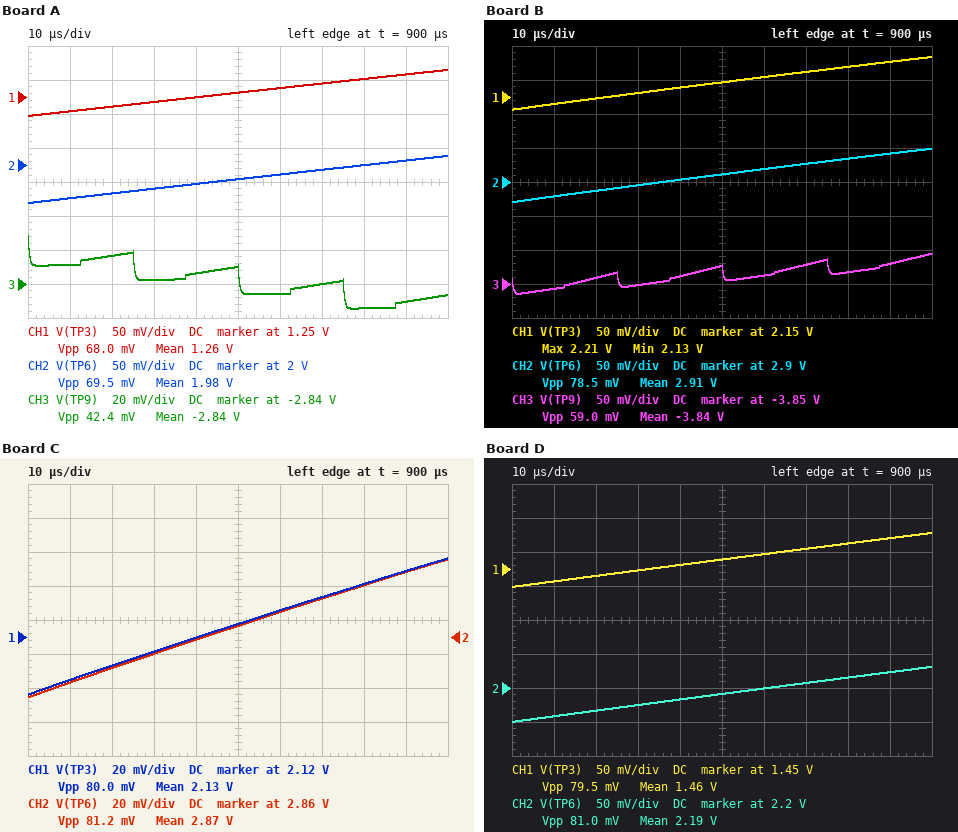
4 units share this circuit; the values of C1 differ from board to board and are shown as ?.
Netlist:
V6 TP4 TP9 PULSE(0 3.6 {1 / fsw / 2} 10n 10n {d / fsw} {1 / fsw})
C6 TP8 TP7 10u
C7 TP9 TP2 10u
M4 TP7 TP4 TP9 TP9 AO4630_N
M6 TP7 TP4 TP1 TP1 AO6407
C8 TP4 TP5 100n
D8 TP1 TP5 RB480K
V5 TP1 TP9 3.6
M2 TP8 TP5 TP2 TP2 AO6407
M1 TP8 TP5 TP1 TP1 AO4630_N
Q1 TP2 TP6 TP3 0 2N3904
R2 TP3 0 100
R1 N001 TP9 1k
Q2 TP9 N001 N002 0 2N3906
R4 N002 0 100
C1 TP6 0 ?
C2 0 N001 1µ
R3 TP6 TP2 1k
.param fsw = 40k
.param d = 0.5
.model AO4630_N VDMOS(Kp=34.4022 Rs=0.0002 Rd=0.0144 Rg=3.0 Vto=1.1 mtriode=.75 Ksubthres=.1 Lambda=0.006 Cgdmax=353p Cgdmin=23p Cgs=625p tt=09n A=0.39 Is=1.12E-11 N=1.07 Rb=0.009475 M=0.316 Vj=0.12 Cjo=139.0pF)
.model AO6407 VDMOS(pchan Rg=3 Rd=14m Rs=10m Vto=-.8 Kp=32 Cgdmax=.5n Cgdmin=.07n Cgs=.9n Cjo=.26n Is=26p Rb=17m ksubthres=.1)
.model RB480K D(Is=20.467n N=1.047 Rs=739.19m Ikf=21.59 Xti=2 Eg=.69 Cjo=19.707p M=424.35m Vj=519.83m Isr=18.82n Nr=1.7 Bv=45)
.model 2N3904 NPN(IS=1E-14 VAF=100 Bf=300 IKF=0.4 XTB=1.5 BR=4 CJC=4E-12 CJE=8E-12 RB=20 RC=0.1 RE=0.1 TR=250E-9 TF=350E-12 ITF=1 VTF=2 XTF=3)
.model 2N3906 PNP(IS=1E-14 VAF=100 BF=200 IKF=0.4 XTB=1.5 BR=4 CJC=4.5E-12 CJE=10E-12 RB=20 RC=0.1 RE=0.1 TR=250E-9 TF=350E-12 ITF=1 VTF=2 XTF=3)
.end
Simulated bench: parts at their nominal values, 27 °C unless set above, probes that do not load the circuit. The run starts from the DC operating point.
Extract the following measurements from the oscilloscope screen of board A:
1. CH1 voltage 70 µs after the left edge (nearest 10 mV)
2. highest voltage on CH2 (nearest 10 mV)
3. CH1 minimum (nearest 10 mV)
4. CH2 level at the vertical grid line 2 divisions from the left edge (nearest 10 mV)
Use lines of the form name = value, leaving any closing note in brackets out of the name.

CH1 voltage 70 µs after the left edge = 1.27 V
highest voltage on CH2 = 2.01 V
CH1 minimum = 1.22 V
CH2 level at the vertical grid line 2 divisions from the left edge = 1.96 V
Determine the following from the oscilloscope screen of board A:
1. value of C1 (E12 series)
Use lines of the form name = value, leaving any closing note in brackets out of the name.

value of C1 = 3.3 µF
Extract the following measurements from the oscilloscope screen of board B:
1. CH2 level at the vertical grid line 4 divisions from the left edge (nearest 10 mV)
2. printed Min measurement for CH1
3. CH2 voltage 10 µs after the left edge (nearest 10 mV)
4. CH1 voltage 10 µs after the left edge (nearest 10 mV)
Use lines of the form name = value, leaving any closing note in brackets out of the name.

CH2 level at the vertical grid line 4 divisions from the left edge = 2.90 V
printed Min measurement for CH1 = 2.13 V
CH2 voltage 10 µs after the left edge = 2.88 V
CH1 voltage 10 µs after the left edge = 2.14 V
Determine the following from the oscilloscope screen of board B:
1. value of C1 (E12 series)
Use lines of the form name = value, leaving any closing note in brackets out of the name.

value of C1 = 390 nF
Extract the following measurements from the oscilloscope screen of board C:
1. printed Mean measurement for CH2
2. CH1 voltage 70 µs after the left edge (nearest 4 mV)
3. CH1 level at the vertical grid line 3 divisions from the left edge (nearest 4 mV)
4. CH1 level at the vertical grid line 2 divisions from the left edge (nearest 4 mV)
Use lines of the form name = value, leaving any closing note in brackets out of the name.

printed Mean measurement for CH2 = 2.87 V
CH1 voltage 70 µs after the left edge = 2.144 V
CH1 level at the vertical grid line 3 divisions from the left edge = 2.112 V
CH1 level at the vertical grid line 2 divisions from the left edge = 2.104 V
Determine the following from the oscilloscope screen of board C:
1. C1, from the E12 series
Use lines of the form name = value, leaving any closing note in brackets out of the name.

C1, from the E12 series = 470 nF
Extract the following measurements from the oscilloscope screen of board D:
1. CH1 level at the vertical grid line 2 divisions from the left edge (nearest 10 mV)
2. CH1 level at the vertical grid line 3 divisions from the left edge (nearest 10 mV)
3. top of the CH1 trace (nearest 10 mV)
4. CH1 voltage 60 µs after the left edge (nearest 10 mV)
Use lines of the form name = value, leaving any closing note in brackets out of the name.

CH1 level at the vertical grid line 2 divisions from the left edge = 1.44 V
CH1 level at the vertical grid line 3 divisions from the left edge = 1.45 V
top of the CH1 trace = 1.50 V
CH1 voltage 60 µs after the left edge = 1.47 V
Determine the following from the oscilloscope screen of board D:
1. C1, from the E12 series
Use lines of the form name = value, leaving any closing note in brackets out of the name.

C1, from the E12 series = 2.2 µF
